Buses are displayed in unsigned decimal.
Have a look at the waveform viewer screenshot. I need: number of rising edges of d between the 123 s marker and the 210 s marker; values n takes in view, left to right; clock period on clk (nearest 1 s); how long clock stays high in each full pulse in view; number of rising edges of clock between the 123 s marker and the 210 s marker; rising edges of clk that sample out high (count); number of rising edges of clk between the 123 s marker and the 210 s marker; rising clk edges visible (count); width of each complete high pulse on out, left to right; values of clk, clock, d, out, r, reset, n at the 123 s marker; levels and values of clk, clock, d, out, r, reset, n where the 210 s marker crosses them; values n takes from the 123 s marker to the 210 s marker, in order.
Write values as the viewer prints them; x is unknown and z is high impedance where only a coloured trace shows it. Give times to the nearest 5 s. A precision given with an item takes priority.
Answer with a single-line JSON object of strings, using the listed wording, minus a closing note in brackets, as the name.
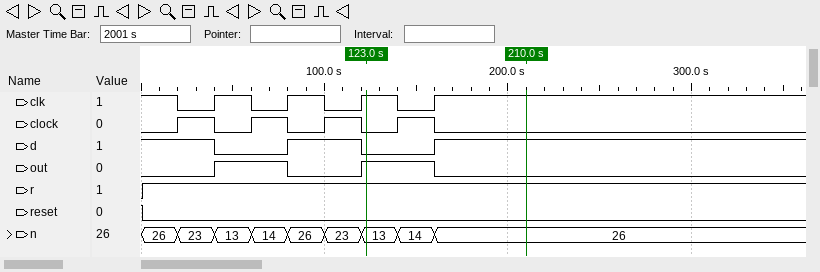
{"number of rising edges of d between the 123 s marker and the 210 s marker": "1", "values n takes in view, left to right": "26, 23, 13, 14, 26, 23, 13, 14, 26", "clock period on clk": "40 s", "how long clock stays high in each full pulse in view": "20 s, 20 s, 20 s, 20 s", "number of rising edges of clock between the 123 s marker and the 210 s marker": "1", "rising edges of clk that sample out high": "2", "number of rising edges of clk between the 123 s marker and the 210 s marker": "1", "rising clk edges visible": "4", "width of each complete high pulse on out, left to right": "40 s, 40 s", "values of clk, clock, d, out, r, reset, n at the 123 s marker": "clk=1, clock=0, d=0, out=1, r=1, reset=0, n=13", "levels and values of clk, clock, d, out, r, reset, n where the 210 s marker crosses them": "clk=1, clock=0, d=1, out=0, r=1, reset=0, n=26", "values n takes from the 123 s marker to the 210 s marker, in order": "13, 14, 26"}
